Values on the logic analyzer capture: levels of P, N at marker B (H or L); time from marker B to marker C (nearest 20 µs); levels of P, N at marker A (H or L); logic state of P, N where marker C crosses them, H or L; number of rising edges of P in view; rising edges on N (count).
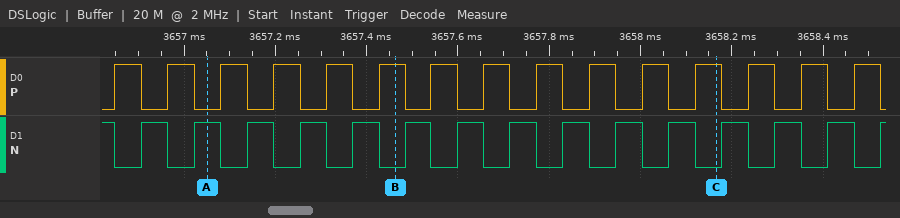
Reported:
P=H, N=L
700 µs
P=L, N=H
P=H, N=L
15
15
